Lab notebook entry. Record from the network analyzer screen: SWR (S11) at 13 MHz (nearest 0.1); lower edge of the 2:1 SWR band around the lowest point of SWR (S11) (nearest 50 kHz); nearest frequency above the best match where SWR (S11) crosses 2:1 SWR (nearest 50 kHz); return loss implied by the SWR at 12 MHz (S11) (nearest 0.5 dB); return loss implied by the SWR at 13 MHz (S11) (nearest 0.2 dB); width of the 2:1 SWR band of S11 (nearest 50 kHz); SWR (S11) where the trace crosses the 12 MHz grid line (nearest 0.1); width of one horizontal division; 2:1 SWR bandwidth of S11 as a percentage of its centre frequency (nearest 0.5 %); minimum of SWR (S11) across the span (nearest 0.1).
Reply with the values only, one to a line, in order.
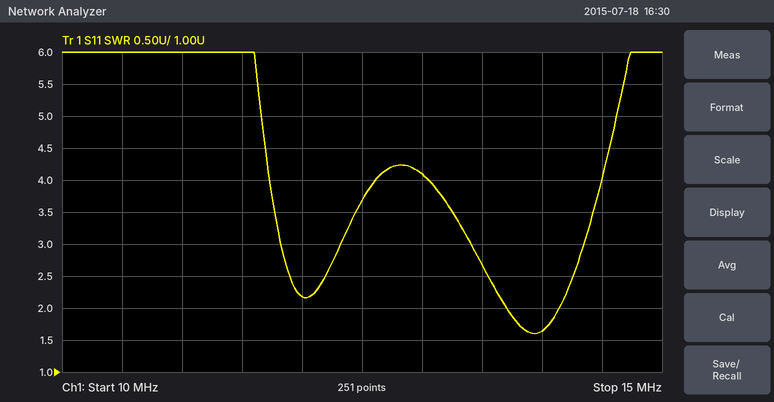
4.1
13.70 MHz
14.15 MHz
8.5 dB
4.4 dB
450 kHz
2.2
500 kHz
3.0 %
1.6
